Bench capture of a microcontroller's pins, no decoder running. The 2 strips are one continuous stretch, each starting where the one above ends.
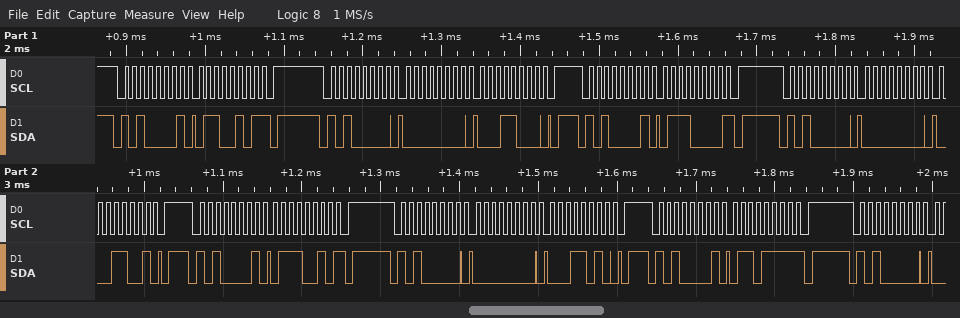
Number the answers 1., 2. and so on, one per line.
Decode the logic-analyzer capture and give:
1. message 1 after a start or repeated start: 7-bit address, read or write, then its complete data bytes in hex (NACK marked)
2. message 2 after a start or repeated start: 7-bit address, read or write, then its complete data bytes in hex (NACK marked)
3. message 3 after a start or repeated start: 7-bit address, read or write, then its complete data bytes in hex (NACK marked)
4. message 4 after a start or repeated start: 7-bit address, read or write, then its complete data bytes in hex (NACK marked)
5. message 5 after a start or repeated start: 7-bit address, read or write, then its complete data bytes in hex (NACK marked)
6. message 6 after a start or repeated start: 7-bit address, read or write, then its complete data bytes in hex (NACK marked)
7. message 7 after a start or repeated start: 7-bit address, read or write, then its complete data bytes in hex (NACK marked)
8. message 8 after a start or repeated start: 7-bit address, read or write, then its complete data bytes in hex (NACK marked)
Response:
1. 0x50 read: 65 NACK
2. 0x50 write: 00 18
3. 0x50 read: 70 NACK
4. 0x50 write: 00 19
5. 0x50 read: 72 NACK
6. 0x50 write: 00 1A
7. 0x50 read: 6F NACK
8. 0x50 write
